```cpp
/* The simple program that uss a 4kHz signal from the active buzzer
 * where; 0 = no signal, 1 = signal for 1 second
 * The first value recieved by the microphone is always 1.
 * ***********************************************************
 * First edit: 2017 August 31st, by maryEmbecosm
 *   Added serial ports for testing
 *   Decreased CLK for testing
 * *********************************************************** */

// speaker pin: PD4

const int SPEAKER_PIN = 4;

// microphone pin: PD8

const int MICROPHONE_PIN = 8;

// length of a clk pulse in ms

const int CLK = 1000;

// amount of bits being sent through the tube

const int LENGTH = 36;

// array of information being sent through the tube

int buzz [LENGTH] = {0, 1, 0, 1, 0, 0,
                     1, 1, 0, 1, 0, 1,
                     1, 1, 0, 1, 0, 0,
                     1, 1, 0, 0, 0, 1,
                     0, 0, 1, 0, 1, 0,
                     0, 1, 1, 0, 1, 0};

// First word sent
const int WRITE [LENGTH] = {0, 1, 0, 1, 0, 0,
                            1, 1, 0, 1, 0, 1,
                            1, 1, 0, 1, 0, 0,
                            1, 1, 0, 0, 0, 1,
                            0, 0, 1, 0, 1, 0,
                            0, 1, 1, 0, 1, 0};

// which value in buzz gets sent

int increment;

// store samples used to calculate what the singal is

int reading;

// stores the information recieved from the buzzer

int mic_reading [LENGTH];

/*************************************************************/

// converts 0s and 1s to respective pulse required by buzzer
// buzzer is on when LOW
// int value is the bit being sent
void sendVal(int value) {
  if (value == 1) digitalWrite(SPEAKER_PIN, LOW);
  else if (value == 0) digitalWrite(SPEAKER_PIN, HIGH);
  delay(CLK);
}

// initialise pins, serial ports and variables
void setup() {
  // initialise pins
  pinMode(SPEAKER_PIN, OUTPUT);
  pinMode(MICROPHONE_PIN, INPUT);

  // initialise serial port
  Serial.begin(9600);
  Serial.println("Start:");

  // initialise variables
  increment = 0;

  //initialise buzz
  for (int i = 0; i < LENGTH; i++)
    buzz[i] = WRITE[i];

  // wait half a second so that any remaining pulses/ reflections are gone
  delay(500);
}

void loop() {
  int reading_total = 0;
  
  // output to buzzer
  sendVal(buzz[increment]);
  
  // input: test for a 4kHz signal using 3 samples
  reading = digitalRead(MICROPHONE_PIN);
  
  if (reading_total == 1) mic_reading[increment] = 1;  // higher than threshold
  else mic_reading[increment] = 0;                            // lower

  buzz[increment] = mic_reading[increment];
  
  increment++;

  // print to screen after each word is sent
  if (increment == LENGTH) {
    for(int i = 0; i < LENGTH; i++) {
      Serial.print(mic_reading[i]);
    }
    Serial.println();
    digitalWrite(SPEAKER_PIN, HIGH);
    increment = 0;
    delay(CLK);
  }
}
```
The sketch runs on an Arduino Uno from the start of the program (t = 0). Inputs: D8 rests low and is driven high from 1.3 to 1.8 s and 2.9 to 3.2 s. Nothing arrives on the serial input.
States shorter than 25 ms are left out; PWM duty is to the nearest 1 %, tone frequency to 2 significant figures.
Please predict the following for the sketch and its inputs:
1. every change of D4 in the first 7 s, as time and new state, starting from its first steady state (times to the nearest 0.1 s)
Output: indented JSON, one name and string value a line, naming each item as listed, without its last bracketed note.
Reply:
{
  "every change of D4 in the first 7 s, as time and new state, starting from its first steady state": "0 s low; 0.5 s high; 1.5 s low; 2.5 s high; 3.5 s low; 4.5 s high; 6.5 s low"
}
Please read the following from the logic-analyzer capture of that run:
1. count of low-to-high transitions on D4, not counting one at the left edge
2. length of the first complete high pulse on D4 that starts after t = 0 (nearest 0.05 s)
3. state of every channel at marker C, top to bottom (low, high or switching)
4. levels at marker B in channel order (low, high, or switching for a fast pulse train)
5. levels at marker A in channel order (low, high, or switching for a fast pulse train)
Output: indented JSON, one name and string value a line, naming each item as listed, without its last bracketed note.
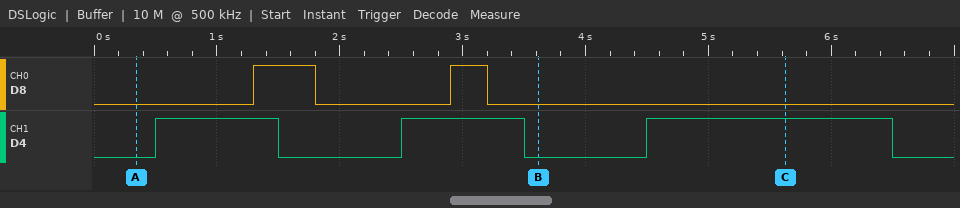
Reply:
{
  "count of low-to-high transitions on D4, not counting one at the left edge": "3",
  "length of the first complete high pulse on D4 that starts after t = 0": "1.00 s",
  "state of every channel at marker C, top to bottom": "D8 low, D4 high",
  "levels at marker B in channel order": "D8 low, D4 low",
  "levels at marker A in channel order": "D8 low, D4 low"
}
